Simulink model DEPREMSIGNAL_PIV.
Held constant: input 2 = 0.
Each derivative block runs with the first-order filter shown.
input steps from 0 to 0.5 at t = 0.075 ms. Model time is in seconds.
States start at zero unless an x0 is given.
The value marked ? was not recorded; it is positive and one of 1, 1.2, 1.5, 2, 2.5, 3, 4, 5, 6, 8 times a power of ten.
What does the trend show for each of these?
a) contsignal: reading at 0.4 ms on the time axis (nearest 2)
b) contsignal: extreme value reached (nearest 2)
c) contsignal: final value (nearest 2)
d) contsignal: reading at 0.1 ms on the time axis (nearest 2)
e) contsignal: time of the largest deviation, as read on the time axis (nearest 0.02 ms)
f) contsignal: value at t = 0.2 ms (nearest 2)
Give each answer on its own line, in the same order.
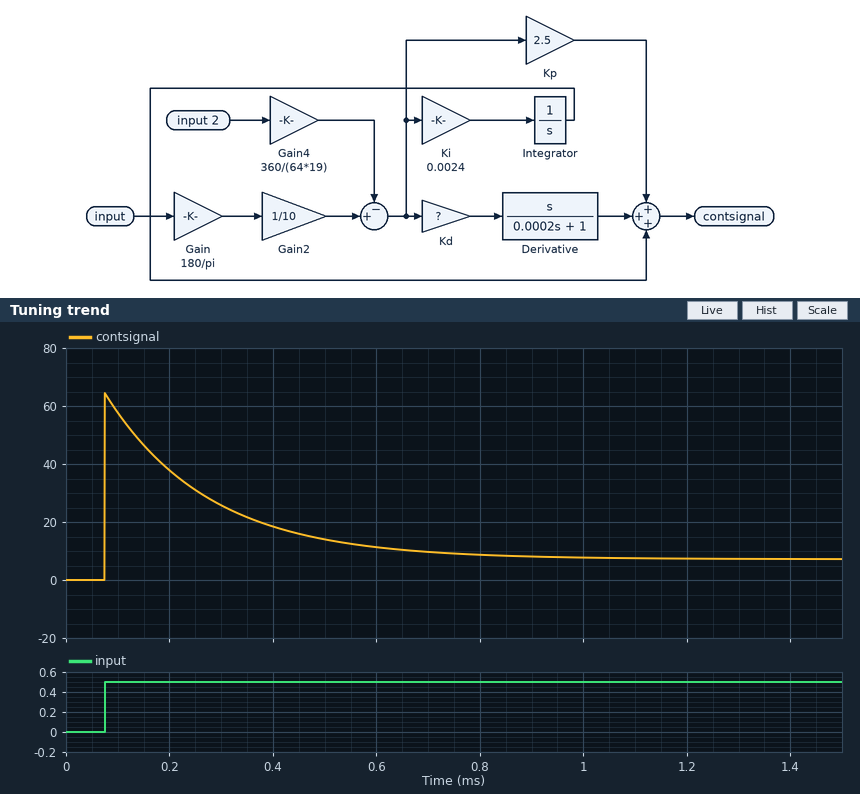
18
64
8
58
0.08 ms
38
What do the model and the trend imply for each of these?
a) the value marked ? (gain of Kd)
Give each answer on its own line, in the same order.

0.004
